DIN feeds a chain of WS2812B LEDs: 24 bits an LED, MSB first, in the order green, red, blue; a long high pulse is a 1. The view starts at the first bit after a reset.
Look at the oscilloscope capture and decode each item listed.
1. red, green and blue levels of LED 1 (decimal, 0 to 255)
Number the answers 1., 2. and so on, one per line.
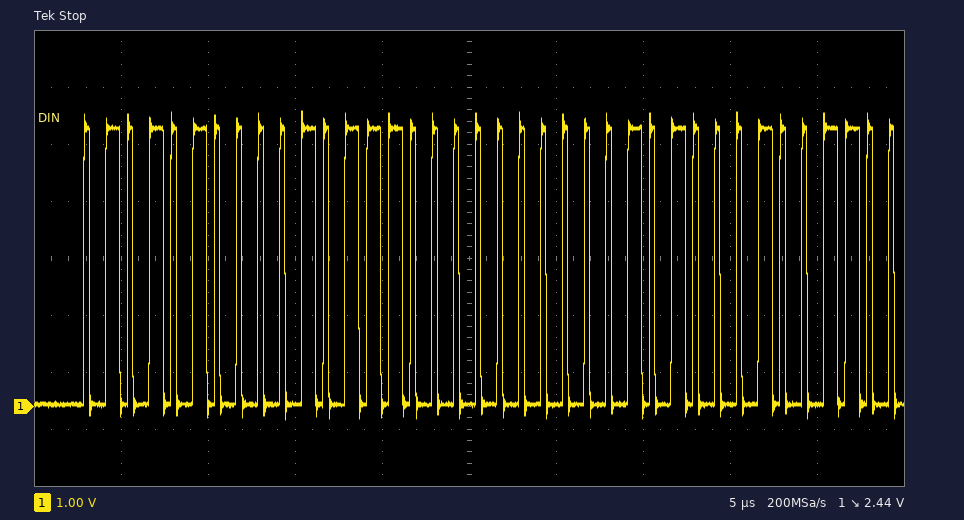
1. 46, 84, 0
